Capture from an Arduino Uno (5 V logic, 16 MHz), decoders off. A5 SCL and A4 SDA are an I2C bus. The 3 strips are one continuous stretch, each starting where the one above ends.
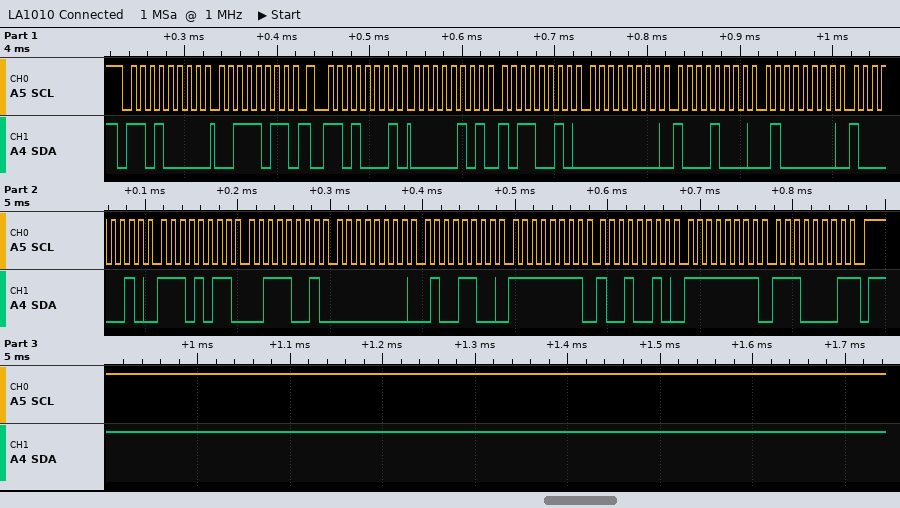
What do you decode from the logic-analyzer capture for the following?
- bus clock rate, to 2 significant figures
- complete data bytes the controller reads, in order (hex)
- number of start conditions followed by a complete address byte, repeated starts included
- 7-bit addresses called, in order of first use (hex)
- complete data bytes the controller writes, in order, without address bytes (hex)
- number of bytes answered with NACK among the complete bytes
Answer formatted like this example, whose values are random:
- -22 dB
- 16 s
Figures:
- 100 kHz
- 05 B2 00 88 40 82 EB 39 00 4C FF 92 FF E1
- 2
- 0x68
- 3B
- 1
